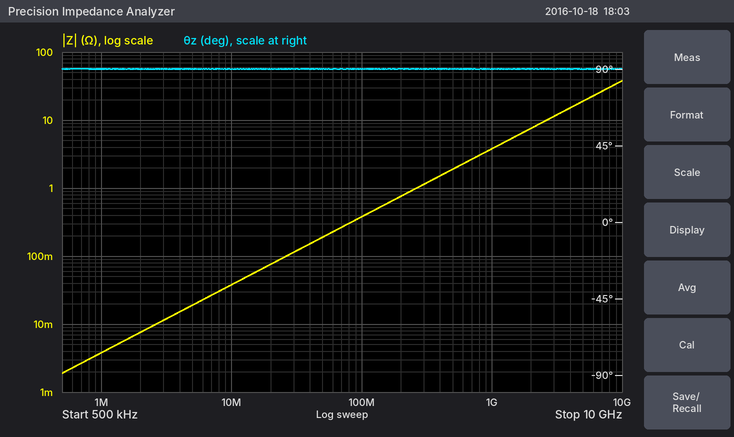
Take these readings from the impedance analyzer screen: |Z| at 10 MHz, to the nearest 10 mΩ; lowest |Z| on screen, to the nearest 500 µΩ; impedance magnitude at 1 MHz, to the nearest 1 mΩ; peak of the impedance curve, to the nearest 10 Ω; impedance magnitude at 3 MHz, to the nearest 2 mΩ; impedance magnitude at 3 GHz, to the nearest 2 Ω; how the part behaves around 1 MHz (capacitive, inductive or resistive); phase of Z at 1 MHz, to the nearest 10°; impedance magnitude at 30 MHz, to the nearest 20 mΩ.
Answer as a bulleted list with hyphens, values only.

- 40 mΩ
- 2.0 mΩ
- 4 mΩ
- 40 Ω
- 12 mΩ
- 12 Ω
- inductive
- 90°
- 120 mΩ
